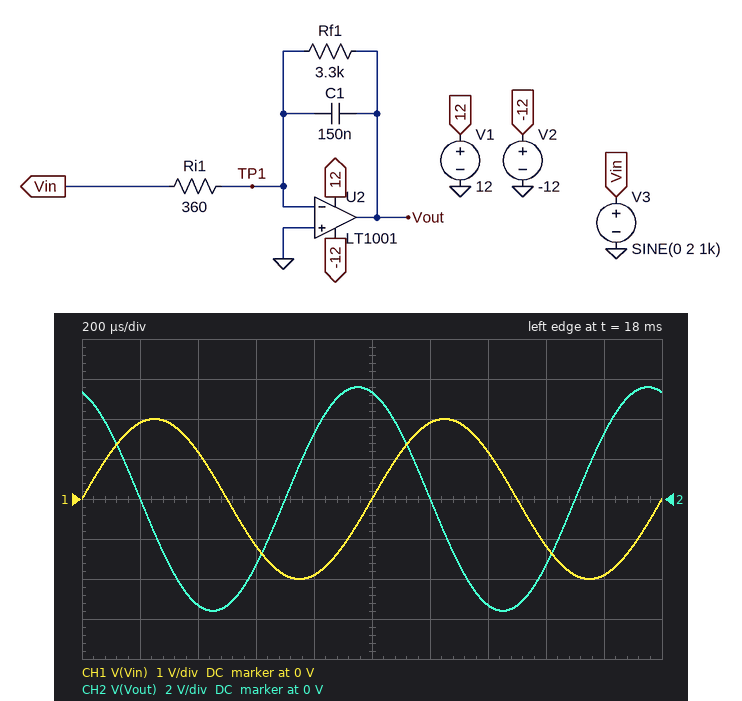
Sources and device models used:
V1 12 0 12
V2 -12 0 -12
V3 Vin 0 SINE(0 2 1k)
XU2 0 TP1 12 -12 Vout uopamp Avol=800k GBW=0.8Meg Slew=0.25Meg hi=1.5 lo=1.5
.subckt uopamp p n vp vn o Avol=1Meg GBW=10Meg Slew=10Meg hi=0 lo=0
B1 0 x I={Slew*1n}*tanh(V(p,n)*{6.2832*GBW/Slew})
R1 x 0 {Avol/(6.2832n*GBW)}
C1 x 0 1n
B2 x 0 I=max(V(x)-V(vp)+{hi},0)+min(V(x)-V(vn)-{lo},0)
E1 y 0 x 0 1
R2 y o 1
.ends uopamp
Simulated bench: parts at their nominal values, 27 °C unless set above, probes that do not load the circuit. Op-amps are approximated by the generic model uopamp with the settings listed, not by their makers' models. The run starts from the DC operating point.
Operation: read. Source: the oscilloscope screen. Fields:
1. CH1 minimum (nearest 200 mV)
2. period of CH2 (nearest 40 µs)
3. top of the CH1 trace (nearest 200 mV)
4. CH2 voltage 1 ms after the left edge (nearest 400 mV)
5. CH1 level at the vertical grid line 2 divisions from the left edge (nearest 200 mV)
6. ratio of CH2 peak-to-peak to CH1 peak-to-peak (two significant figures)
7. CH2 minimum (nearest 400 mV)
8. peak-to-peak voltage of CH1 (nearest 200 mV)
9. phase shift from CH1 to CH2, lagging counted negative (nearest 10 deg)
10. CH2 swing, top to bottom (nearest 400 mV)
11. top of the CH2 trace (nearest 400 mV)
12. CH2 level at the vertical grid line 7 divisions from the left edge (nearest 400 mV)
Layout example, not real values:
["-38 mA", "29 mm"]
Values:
["-2.0 V", "1.00 ms", "2.0 V", "5.2 V", "1.2 V", "2.8", "-5.6 V", "4.0 V", "110 deg", "11.2 V", "5.6 V", "-5.2 V"]
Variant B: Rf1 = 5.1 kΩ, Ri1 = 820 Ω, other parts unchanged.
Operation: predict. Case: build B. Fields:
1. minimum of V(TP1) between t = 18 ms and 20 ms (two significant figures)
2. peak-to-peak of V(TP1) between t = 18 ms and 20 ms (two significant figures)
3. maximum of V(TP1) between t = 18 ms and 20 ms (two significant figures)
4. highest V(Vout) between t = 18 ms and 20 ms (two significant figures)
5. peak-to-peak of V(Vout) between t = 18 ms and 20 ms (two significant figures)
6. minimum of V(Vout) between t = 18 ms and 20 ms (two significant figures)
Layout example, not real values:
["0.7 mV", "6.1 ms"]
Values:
["-3.2 mV", "6.3 mV", "3.2 mV", "2.5 V", "5.1 V", "-2.5 V"]
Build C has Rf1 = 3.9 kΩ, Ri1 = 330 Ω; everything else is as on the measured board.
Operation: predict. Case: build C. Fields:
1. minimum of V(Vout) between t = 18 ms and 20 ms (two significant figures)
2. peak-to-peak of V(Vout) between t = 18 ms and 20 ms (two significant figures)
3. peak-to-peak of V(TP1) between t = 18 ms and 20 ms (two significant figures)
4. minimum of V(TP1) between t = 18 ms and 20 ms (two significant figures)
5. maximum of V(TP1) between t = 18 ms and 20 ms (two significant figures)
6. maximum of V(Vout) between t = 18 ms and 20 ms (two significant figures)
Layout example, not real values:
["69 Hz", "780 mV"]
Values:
["-6.2 V", "12 V", "16 mV", "-7.8 mV", "7.8 mV", "6.2 V"]
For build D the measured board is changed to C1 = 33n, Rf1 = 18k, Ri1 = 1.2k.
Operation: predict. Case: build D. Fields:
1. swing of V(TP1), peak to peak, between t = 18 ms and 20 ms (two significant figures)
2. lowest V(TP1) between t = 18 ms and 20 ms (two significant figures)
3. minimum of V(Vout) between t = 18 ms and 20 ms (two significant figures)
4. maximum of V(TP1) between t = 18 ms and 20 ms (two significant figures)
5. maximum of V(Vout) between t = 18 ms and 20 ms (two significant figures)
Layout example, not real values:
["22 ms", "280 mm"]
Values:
["20 mV", "-9.8 mV", "-7.7 V", "9.8 mV", "7.7 V"]
